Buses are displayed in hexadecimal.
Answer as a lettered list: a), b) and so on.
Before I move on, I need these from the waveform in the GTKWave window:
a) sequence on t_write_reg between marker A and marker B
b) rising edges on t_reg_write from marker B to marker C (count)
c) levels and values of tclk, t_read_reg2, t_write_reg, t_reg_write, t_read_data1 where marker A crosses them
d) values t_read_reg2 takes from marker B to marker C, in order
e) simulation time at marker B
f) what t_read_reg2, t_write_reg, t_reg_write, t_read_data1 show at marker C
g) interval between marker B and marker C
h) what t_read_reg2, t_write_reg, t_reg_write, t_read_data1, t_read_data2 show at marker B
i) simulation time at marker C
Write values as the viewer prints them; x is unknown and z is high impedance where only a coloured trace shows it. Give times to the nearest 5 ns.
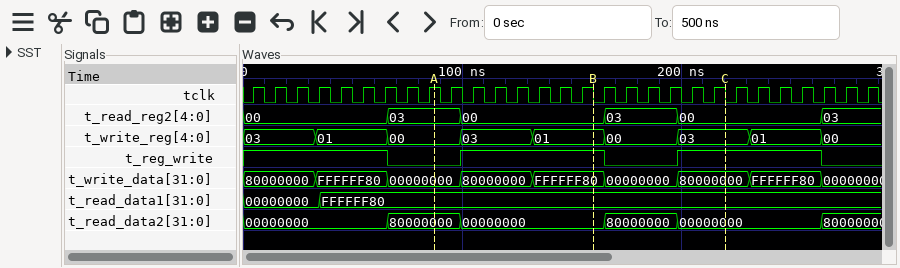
a) 00, 03, 01
b) 1
c) tclk=1, t_read_reg2=03, t_write_reg=00, t_reg_write=0, t_read_data1=FFFFFF80
d) 00, 03, 00
e) 160 ns
f) t_read_reg2=00, t_write_reg=03, t_reg_write=1, t_read_data1=FFFFFF80
g) 60 ns
h) t_read_reg2=00, t_write_reg=01, t_reg_write=1, t_read_data1=FFFFFF80, t_read_data2=00000000
i) 220 ns
